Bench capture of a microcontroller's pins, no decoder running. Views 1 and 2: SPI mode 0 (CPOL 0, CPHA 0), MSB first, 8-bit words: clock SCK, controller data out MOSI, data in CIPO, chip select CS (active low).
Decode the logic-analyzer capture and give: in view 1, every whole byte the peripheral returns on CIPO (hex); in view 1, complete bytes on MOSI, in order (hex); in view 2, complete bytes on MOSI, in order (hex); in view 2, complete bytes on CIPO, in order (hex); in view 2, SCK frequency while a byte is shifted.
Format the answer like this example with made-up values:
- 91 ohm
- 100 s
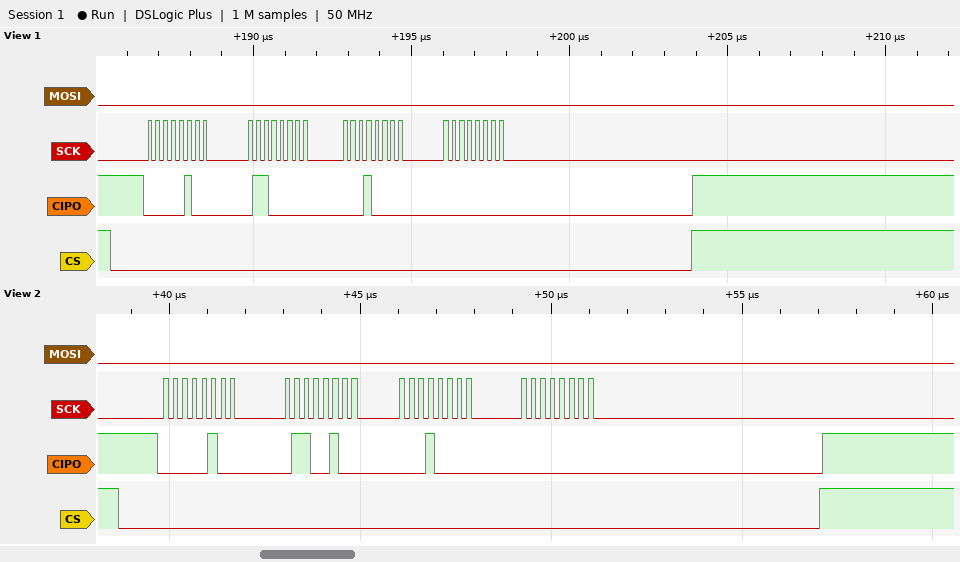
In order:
- 04 60 10 00
- 00 00 00 00
- 00 00 00 00
- 04 64 10 00
- 4 MHz
